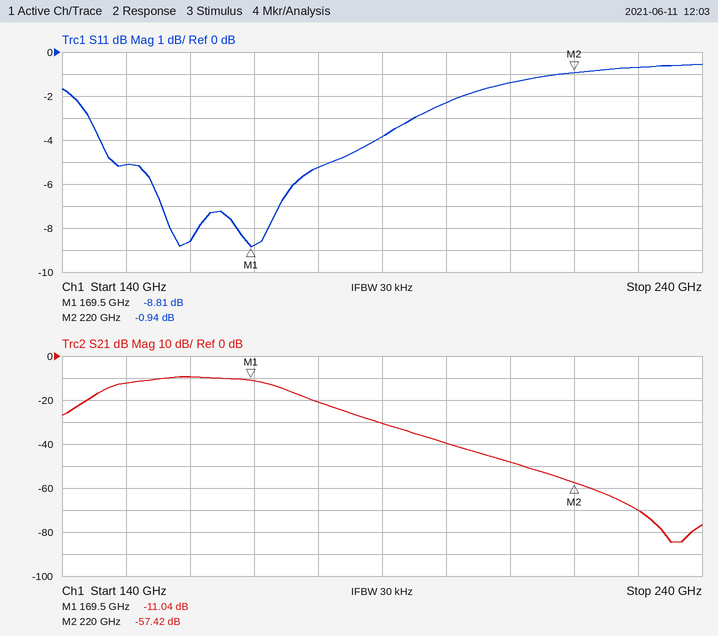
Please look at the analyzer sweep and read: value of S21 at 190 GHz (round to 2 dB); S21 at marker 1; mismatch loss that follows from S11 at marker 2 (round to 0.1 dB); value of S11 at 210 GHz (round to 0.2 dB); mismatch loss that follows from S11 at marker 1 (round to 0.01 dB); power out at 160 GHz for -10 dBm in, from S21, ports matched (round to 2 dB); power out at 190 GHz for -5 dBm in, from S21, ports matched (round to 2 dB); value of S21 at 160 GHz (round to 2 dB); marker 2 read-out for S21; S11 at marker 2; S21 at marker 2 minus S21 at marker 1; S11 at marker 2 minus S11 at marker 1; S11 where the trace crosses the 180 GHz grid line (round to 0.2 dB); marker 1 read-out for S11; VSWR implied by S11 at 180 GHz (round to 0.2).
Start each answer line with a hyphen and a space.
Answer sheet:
- -30 dB
- -11.04 dB
- 7.1 dB
- -1.4 dB
- 0.61 dB
- -20 dBm
- -36 dBm
- -10 dB
- -57.42 dB
- -0.94 dB
- -46.38 dB
- 7.87 dB
- -5.2 dB
- -8.81 dB
- 3.4
